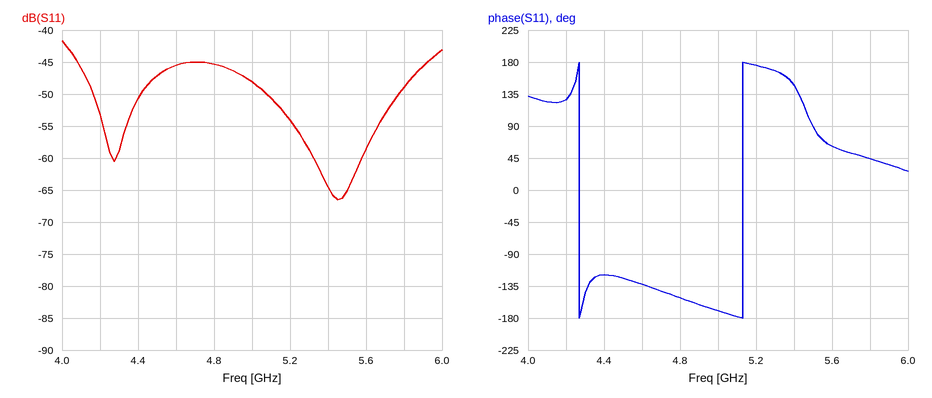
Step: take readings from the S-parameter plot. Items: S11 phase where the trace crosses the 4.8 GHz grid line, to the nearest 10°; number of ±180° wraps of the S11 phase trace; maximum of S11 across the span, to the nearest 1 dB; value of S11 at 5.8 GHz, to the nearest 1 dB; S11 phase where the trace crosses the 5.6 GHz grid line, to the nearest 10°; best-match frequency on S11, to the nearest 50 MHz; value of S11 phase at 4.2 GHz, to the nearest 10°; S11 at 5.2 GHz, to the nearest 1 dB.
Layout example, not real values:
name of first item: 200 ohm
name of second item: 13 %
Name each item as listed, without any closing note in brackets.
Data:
S11 phase where the trace crosses the 4.8 GHz grid line, to the nearest 10°: -150°
number of ±180° wraps of the S11 phase trace: 2
maximum of S11 across the span, to the nearest 1 dB: -42 dB
value of S11 at 5.8 GHz, to the nearest 1 dB: -49 dB
S11 phase where the trace crosses the 5.6 GHz grid line, to the nearest 10°: 60°
best-match frequency on S11, to the nearest 50 MHz: 5.45 GHz
value of S11 phase at 4.2 GHz, to the nearest 10°: 130°
S11 at 5.2 GHz, to the nearest 1 dB: -54 dB
